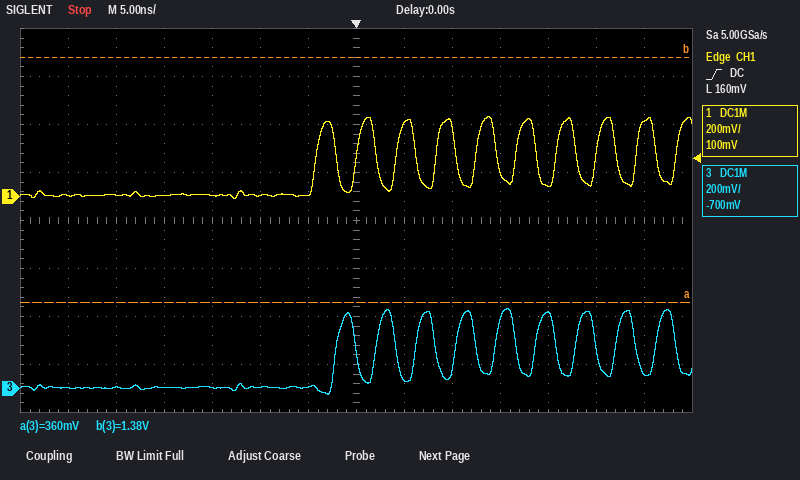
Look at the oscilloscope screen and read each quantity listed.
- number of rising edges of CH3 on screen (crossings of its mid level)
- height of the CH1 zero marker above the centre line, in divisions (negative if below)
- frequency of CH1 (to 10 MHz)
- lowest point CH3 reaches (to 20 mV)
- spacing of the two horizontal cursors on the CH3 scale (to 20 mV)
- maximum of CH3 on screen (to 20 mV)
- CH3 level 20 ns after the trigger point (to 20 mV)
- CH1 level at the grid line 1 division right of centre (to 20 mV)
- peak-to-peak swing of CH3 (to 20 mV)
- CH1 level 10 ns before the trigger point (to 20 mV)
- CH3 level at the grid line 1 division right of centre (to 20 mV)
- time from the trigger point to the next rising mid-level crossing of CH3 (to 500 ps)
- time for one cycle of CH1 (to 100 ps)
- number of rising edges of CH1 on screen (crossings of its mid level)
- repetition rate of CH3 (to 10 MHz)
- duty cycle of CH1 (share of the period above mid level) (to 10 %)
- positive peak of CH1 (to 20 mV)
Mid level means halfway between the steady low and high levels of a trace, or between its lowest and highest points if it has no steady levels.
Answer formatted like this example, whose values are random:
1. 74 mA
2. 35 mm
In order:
1. 9
2. +0.5 div
3. 240 MHz
4. -20 mV
5. 1.02 V
6. 340 mV
7. 320 mV
8. 300 mV
9. 360 mV
10. 0 mV
11. 40 mV
12. 2.0 ns
13. 4.2 ns
14. 10
15. 240 MHz
16. 50 %
17. 340 mV
